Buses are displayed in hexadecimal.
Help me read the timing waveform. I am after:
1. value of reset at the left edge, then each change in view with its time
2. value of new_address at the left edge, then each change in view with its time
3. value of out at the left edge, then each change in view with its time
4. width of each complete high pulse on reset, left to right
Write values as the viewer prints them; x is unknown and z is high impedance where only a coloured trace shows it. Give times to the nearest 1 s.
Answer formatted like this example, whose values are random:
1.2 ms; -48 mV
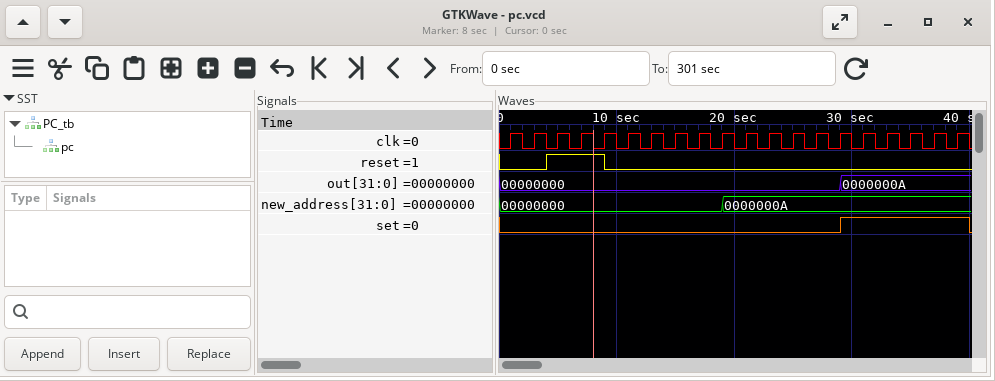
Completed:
0, 1 at 4 s, 0 at 9 s; 00000000, 0000000A at 19 s; 00000000, 0000000A at 29 s; 5 s
